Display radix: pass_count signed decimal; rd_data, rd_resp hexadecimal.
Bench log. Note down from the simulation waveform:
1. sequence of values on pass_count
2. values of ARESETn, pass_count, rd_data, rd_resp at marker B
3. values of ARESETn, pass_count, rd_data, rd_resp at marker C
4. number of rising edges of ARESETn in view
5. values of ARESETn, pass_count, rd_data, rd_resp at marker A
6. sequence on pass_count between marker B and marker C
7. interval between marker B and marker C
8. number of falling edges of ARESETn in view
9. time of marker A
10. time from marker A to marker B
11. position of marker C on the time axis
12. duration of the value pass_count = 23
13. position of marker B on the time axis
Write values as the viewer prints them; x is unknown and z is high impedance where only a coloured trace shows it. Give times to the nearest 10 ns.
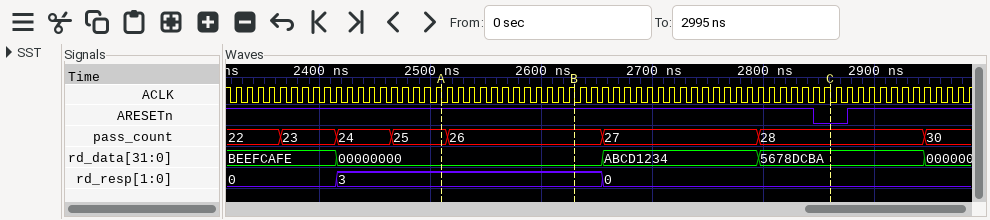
22, 23, 24, 25, 26, 27, 28, 30
ARESETn=1, pass_count=26, rd_data=00000000, rd_resp=3
ARESETn=0, pass_count=28, rd_data=5678DCBA, rd_resp=0
1
ARESETn=1, pass_count=25, rd_data=00000000, rd_resp=3
26, 27, 28
230 ns
1
2510 ns
120 ns
2860 ns
50 ns
2630 ns
